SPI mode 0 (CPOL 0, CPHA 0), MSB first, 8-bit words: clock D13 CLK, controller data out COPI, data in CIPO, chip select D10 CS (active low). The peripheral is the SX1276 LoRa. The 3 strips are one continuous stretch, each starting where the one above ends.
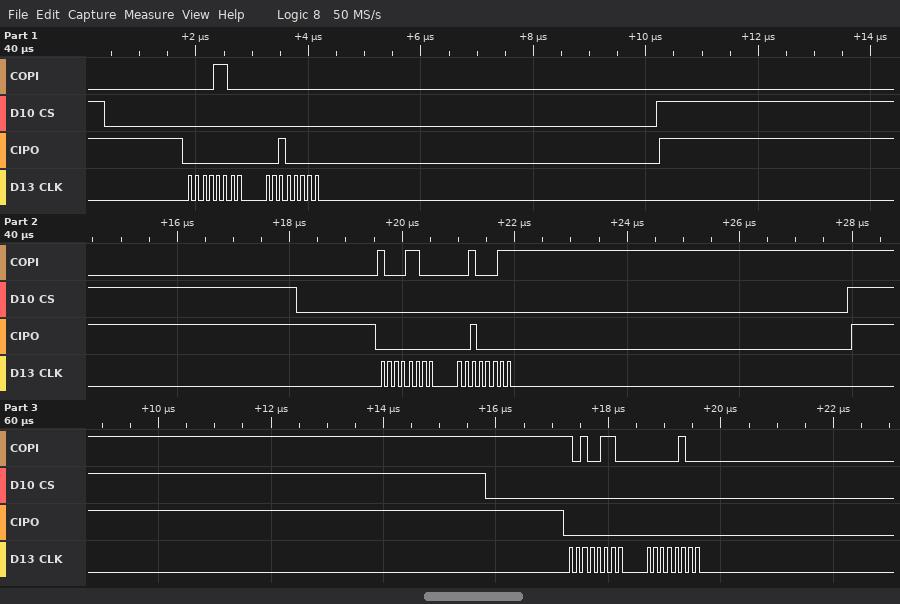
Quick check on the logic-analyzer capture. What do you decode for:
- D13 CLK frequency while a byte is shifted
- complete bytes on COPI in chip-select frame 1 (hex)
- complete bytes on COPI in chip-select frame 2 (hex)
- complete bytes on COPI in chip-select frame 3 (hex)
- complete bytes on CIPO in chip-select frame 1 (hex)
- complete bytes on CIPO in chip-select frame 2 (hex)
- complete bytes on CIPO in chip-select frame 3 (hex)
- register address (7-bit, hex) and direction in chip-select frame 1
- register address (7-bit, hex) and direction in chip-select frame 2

8 MHz
0C 00
8C 23
A6 04
00 20
00 20
00 00
0x0C read
0x0C write
